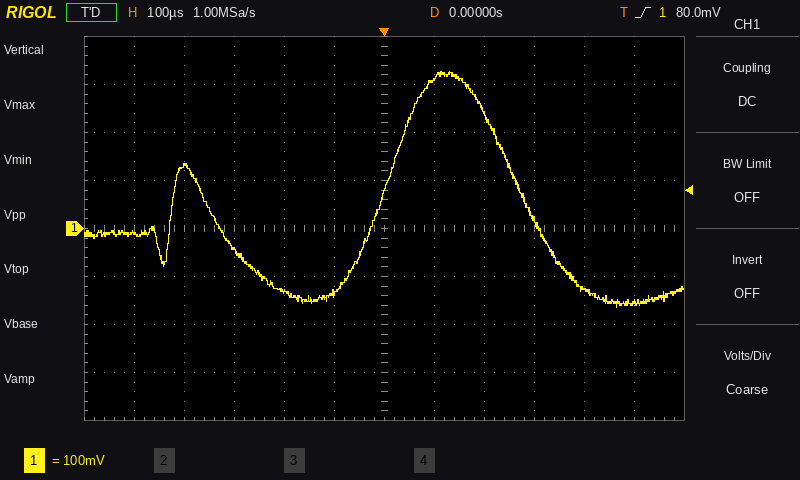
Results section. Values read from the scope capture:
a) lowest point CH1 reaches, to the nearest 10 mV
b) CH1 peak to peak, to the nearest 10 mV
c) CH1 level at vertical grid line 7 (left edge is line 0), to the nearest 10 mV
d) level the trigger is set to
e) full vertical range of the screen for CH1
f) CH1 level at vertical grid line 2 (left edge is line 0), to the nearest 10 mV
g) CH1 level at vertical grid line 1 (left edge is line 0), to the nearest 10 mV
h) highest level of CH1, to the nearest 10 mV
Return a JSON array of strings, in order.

["-160 mV", "490 mV", "310 mV", "80.0 mV", "800 mV", "130 mV", "-10 mV", "330 mV"]
